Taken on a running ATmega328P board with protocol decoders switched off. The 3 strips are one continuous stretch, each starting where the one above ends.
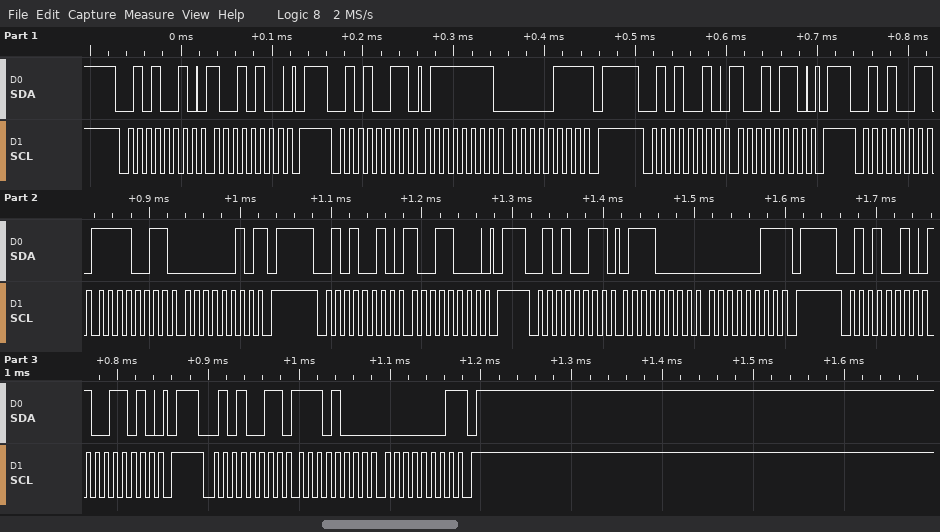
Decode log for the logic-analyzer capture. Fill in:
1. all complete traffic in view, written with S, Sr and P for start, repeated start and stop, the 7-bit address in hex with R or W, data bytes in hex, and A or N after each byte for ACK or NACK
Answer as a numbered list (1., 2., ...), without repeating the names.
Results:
1. S 29W A 94 A P S 29R A 7F A 07 N P S 29W A 96 A P S 29R A F3 A 02 N P S 29W A 98 A P S 29R A 70 A 03 N P S 29W A 9A A P S 29R A E8 A 01 N P
